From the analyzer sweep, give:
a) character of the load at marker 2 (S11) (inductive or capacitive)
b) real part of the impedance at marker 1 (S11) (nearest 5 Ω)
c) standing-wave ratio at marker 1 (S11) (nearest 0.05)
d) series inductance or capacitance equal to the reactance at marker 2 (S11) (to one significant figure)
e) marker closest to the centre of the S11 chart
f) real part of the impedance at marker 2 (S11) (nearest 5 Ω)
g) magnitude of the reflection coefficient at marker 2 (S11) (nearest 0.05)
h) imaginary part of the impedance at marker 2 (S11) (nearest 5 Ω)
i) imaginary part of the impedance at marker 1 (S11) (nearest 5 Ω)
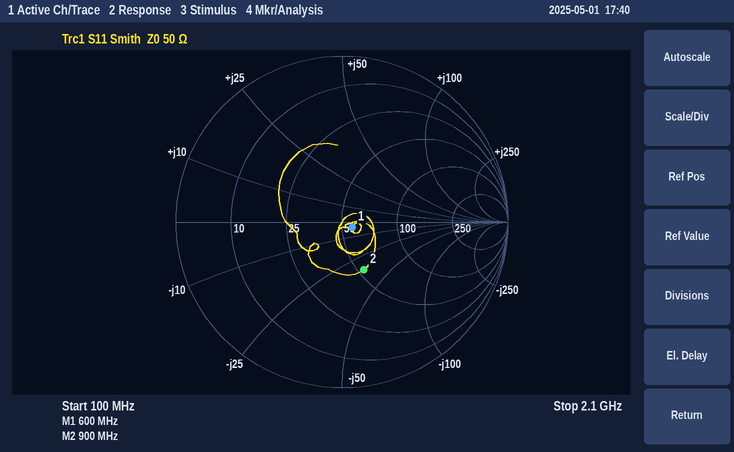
capacitive
55 Ω
1.15
5 pF
marker 1
55 Ω
0.30
-35 Ω
-5 Ω
